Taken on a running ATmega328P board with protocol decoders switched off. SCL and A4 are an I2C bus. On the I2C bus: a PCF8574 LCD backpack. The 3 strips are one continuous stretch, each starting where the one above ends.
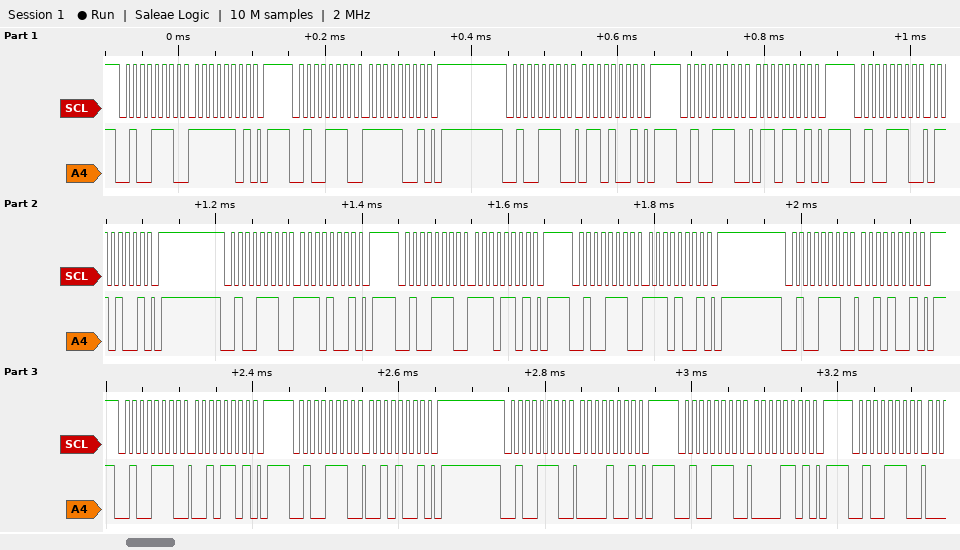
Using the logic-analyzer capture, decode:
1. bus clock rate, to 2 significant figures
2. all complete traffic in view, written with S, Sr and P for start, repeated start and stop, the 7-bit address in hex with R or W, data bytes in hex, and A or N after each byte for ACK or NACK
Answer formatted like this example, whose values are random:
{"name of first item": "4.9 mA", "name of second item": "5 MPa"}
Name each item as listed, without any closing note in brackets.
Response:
{"bus clock rate, to 2 significant figures": "100 kHz", "all complete traffic in view, written with S, Sr and P for start, repeated start and stop, the 7-bit address in hex with R or W, data bytes in hex, and A or N after each byte for ACK or NACK": "S 27W A FD A P S 27W A F9 A P S 27W A 69 A P S 27W A 6D A P S 27W A 69 A P S 27W A E9 A P S 27W A ED A P S 27W A E9 A P S 27W A 29 A P S 27W A 2D A P S 27W A 29 A P S 27W A 09 A P S 27W A 0D A P S 27W A"}
